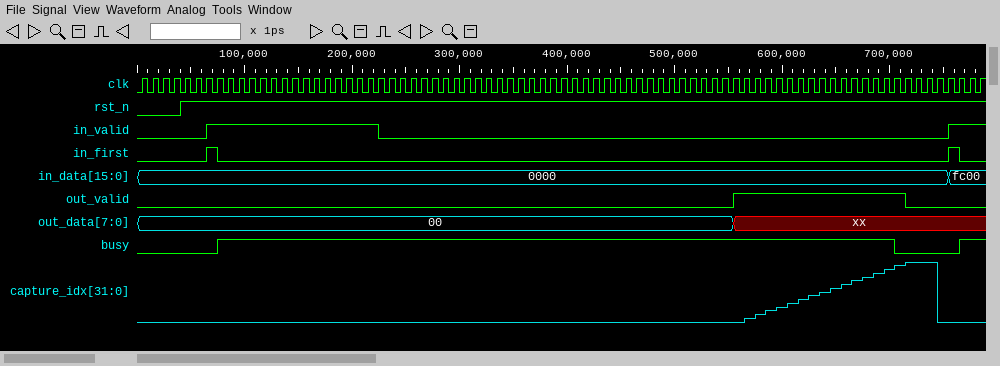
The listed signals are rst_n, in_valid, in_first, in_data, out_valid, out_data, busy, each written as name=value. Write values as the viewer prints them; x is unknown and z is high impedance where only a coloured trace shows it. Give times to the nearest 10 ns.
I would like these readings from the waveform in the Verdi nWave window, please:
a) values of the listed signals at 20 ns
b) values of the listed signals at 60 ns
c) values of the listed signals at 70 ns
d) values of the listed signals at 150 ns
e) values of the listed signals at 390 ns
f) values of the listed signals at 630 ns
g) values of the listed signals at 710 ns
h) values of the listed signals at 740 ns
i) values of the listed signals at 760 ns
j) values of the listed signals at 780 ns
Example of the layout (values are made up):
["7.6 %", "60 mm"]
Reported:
["rst_n=0, in_valid=0, in_first=0, in_data=0000, out_valid=0, out_data=00, busy=0", "rst_n=1, in_valid=0, in_first=0, in_data=0000, out_valid=0, out_data=00, busy=0", "rst_n=1, in_valid=1, in_first=1, in_data=0000, out_valid=0, out_data=00, busy=0", "rst_n=1, in_valid=1, in_first=0, in_data=0000, out_valid=0, out_data=00, busy=1", "rst_n=1, in_valid=0, in_first=0, in_data=0000, out_valid=0, out_data=00, busy=1", "rst_n=1, in_valid=0, in_first=0, in_data=0000, out_valid=1, out_data=xx, busy=1", "rst_n=1, in_valid=0, in_first=0, in_data=0000, out_valid=1, out_data=xx, busy=0", "rst_n=1, in_valid=0, in_first=0, in_data=0000, out_valid=0, out_data=xx, busy=0", "rst_n=1, in_valid=1, in_first=1, in_data=fc00, out_valid=0, out_data=xx, busy=0", "rst_n=1, in_valid=1, in_first=0, in_data=fc00, out_valid=0, out_data=xx, busy=1"]
